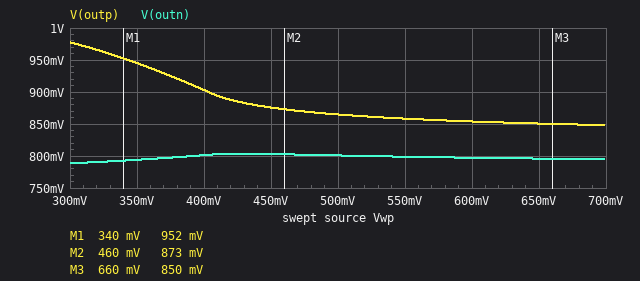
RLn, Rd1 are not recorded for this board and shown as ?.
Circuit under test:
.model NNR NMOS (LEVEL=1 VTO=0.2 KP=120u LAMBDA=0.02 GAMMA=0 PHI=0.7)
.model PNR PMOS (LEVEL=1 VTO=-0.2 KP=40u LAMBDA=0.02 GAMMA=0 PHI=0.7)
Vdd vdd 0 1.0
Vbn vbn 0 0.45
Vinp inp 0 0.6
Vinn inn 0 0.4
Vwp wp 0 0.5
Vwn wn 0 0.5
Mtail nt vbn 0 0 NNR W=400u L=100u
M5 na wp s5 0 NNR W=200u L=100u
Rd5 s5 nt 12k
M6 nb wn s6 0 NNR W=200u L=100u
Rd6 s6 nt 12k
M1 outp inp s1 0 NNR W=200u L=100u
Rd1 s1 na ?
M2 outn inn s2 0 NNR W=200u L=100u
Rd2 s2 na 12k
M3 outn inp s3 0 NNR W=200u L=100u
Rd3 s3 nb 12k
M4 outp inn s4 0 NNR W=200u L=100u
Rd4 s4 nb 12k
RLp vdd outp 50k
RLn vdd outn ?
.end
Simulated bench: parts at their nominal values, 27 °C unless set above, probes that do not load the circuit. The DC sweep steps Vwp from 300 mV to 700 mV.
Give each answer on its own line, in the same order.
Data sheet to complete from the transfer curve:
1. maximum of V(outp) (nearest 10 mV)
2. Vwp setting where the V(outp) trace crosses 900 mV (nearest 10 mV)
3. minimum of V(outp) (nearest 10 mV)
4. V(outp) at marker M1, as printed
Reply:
980 mV
400 mV
850 mV
952 mV
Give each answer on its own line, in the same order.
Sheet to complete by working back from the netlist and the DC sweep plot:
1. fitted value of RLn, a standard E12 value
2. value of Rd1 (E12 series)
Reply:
56 kΩ
33 kΩ
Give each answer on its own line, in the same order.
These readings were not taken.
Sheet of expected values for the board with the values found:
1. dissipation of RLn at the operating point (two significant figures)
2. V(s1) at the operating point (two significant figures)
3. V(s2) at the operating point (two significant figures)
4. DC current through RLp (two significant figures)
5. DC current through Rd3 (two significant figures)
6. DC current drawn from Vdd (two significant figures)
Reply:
710 nW
250 mV
160 mV
2.7 µA
3.4 µA
6.3 µA
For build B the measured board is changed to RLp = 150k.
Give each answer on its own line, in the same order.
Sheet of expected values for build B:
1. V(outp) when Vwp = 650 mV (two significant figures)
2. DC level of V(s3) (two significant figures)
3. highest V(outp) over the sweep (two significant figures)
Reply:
550 mV
230 mV
930 mV
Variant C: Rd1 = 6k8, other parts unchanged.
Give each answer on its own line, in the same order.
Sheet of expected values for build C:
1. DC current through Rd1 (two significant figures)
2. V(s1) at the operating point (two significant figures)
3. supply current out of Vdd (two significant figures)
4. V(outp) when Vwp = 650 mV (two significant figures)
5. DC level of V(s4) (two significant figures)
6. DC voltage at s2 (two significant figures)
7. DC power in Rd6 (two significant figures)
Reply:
3.5 µA
230 mV
6.8 µA
790 mV
200 mV
210 mV
130 nW
